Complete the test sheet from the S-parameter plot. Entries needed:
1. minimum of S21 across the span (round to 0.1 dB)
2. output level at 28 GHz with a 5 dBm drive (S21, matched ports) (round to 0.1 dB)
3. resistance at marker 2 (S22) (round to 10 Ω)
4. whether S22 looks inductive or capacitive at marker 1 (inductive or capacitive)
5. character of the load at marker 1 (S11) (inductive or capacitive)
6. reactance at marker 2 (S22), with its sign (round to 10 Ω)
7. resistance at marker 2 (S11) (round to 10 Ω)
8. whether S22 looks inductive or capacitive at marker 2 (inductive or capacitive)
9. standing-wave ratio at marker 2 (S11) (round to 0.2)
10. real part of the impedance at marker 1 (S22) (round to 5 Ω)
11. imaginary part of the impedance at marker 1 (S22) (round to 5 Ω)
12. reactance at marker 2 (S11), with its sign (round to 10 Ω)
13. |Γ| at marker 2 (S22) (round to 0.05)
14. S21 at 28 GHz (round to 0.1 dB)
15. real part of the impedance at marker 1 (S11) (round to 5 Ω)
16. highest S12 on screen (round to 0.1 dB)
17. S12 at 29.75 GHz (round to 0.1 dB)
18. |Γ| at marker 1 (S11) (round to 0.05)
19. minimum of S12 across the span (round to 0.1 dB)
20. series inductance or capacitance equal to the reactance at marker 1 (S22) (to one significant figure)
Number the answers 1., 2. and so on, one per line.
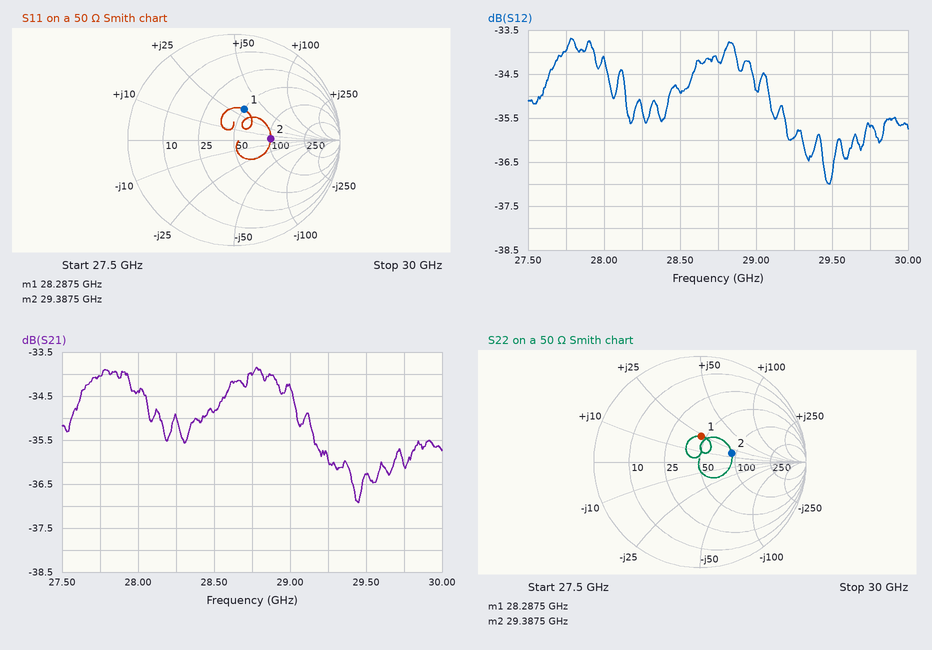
1. -36.9 dB
2. -29.4 dBm
3. 90 Ω
4. inductive
5. inductive
6. +20 Ω
7. 100 Ω
8. inductive
9. 2.0
10. 45 Ω
11. +25 Ω
12. 0 Ω
13. 0.30
14. -34.4 dB
15. 50 Ω
16. -33.7 dB
17. -35.7 dB
18. 0.30
19. -37.0 dB
20. 100 pH
